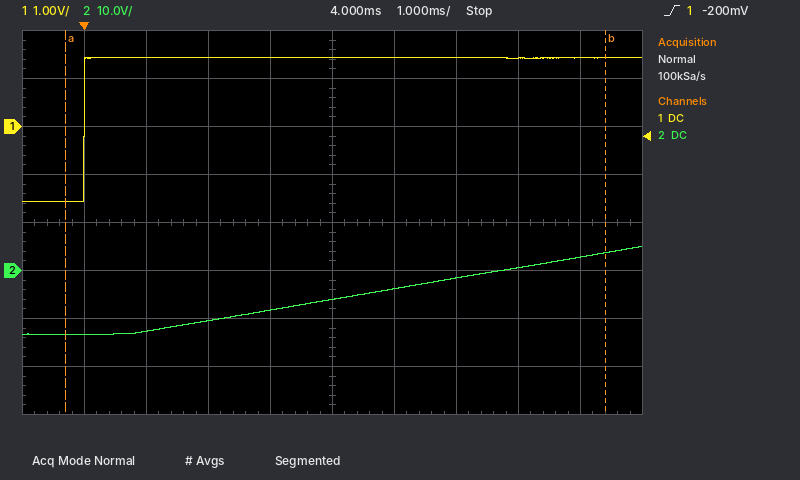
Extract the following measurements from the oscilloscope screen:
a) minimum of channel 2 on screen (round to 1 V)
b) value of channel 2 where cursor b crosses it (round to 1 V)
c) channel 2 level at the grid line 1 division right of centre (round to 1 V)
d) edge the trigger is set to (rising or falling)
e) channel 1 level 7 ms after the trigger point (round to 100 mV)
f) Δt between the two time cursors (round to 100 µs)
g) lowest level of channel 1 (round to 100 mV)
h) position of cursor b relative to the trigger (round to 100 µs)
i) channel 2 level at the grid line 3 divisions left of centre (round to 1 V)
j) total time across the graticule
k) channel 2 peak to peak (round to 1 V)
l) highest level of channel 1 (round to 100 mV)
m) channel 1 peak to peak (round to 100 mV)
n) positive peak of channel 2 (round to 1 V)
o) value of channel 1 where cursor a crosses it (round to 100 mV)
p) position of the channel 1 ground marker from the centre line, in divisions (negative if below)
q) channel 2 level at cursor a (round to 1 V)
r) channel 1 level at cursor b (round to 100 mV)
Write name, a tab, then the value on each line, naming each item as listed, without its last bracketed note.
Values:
minimum of channel 2 on screen	-13 V
value of channel 2 where cursor b crosses it	4 V
channel 2 level at the grid line 1 division right of centre	-4 V
edge the trigger is set to	rising
channel 1 level 7 ms after the trigger point	1.4 V
Δt between the two time cursors	8.7 ms
lowest level of channel 1	-1.6 V
position of cursor b relative to the trigger	+8.4 ms
channel 2 level at the grid line 3 divisions left of centre	-13 V
total time across the graticule	10 ms
channel 2 peak to peak	18 V
highest level of channel 1	1.4 V
channel 1 peak to peak	3.0 V
positive peak of channel 2	5 V
value of channel 1 where cursor a crosses it	-1.6 V
position of the channel 1 ground marker from the centre line, in divisions	+2.0 div
channel 2 level at cursor a	-13 V
channel 1 level at cursor b	1.4 V
